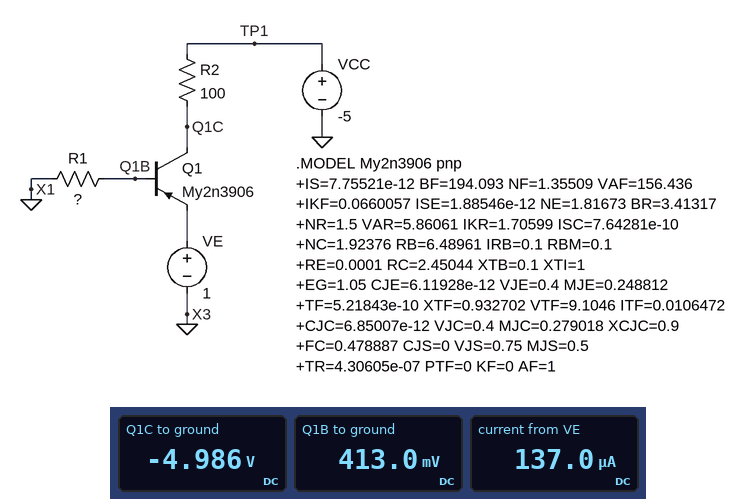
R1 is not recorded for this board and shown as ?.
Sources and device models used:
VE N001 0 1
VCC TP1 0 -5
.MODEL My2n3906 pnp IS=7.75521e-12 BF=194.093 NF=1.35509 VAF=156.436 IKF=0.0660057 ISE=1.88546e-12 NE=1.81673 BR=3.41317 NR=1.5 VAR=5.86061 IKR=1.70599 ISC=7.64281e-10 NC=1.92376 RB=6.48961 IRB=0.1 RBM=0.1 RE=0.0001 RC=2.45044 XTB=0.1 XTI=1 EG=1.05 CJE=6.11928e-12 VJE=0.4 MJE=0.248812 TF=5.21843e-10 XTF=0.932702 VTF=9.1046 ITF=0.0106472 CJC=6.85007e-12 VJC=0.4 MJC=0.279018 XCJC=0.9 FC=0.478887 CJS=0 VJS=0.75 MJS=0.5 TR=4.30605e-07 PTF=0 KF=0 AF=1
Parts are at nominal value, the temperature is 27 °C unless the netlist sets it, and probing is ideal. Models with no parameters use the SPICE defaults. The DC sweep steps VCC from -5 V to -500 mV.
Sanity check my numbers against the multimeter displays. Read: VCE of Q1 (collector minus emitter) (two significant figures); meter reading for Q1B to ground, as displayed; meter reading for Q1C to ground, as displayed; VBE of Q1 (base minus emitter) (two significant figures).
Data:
-6.0 V
413.0 mV
-4.986 V
-590 mV
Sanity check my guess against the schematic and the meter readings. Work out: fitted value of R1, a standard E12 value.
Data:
330 kΩ
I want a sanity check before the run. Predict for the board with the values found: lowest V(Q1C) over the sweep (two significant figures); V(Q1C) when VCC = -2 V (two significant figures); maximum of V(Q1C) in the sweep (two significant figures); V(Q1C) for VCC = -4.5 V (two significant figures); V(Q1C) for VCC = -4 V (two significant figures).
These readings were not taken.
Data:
-5.0 V
-2.0 V
-490 mV
-4.5 V
-4.0 V
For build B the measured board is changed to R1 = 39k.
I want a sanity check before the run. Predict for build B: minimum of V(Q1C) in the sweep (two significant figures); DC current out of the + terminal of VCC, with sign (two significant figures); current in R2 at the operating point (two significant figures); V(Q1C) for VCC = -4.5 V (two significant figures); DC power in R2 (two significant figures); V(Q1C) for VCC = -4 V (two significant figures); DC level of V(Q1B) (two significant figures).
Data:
-4.9 V
-1.1 mA
1.1 mA
-4.4 V
120 µW
-3.9 V
340 mV
